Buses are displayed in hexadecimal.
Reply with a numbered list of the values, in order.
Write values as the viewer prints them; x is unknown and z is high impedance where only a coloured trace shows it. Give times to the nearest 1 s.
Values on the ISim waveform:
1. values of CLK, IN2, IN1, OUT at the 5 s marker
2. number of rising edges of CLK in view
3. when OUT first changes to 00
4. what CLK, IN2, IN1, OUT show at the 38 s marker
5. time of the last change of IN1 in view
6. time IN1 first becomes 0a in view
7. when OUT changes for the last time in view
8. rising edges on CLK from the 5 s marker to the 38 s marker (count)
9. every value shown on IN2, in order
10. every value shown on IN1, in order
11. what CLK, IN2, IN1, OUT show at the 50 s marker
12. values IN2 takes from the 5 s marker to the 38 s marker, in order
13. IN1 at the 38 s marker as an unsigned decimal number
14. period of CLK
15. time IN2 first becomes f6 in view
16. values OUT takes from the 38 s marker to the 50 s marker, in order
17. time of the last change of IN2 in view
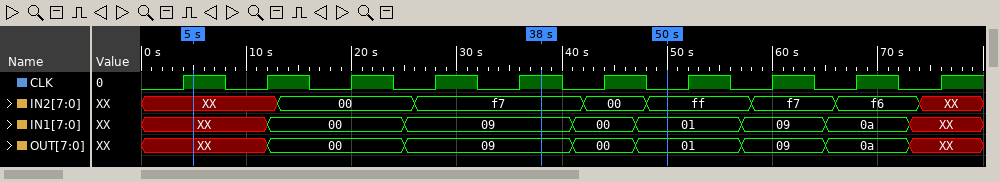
1. CLK=1, IN2=XX, IN1=XX, OUT=XX
2. 10
3. 12 s
4. CLK=1, IN2=f7, IN1=09, OUT=09
5. 73 s
6. 65 s
7. 73 s
8. 4
9. XX, 00, f7, 00, ff, f7, f6, XX
10. XX, 00, 09, 00, 01, 09, 0a, XX
11. CLK=0, IN2=ff, IN1=01, OUT=01
12. XX, 00, f7
13. 9
14. 8 s
15. 66 s
16. 09, 00, 01
17. 74 s
